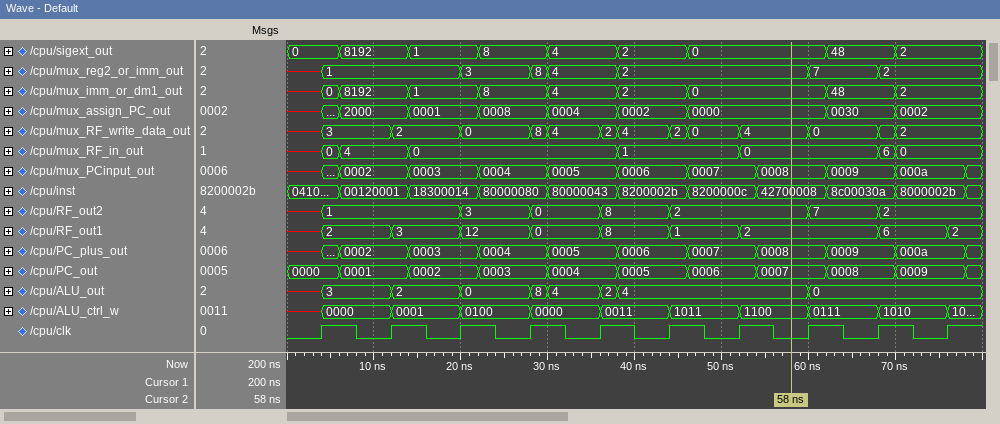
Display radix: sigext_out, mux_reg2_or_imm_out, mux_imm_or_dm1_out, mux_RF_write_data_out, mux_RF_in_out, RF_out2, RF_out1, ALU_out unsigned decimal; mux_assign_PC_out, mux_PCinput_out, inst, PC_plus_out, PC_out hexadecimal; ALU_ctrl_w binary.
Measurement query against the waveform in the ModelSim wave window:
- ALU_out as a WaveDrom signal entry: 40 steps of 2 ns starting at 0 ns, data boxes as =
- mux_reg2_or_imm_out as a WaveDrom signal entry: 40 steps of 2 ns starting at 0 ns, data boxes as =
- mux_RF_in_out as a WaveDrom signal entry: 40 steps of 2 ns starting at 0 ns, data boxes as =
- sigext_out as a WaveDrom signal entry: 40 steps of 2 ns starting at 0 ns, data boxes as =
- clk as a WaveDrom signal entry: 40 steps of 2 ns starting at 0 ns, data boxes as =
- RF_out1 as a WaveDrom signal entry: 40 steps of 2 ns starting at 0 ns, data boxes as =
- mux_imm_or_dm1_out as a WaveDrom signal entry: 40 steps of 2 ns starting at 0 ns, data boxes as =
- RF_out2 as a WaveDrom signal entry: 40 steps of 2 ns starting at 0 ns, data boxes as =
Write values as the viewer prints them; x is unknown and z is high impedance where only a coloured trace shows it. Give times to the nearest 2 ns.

{name: 'ALU_out', wave: 'x.=...=...=...==..==..........=.........', data: '3 2 0 8 4 2 4 0'}
{name: 'mux_reg2_or_imm_out', wave: 'x.=.......=...==...=..........=...=.....', data: '1 3 8 4 2 7 2'}
{name: 'mux_RF_in_out', wave: 'x.==...=...........=......=.......==....', data: '0 4 0 1 0 6 0'}
{name: 'sigext_out', wave: '=..=...=...=...=...=...=.......=...=....', data: '0 8192 1 8 4 2 0 48 2'}
{name: 'clk', wave: '0.1.0.1.0.1.0.1.0.1.0.1.0.1.0.1.0.1.0.1.'}
{name: 'RF_out1', wave: 'x.=...=...=...=...=...=...=.......=...=.', data: '2 3 12 0 8 1 2 6 2'}
{name: 'mux_imm_or_dm1_out', wave: 'x.==...=...=...=...=...=.......=...=....', data: '0 8192 1 8 4 2 0 48 2'}
{name: 'RF_out2', wave: 'x.=.......=...=...=...=.......=...=.....', data: '1 3 0 8 2 7 2'}
